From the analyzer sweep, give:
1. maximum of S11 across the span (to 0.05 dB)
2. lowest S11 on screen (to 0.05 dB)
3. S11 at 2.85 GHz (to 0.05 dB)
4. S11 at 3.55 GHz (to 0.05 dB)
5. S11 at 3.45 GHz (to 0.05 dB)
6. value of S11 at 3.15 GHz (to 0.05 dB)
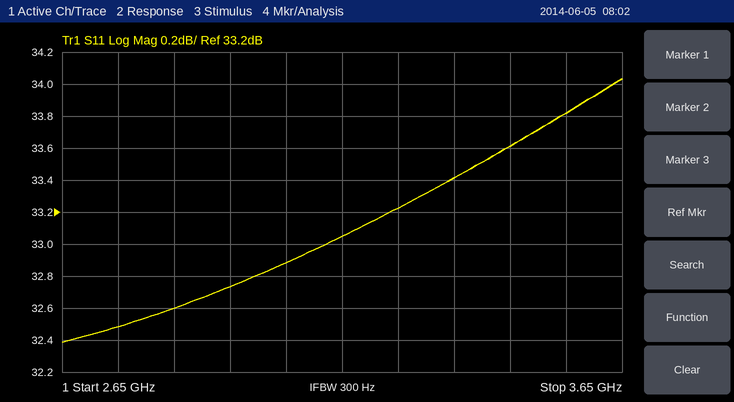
34.05 dB
32.40 dB
32.60 dB
33.80 dB
33.60 dB
33.05 dB
